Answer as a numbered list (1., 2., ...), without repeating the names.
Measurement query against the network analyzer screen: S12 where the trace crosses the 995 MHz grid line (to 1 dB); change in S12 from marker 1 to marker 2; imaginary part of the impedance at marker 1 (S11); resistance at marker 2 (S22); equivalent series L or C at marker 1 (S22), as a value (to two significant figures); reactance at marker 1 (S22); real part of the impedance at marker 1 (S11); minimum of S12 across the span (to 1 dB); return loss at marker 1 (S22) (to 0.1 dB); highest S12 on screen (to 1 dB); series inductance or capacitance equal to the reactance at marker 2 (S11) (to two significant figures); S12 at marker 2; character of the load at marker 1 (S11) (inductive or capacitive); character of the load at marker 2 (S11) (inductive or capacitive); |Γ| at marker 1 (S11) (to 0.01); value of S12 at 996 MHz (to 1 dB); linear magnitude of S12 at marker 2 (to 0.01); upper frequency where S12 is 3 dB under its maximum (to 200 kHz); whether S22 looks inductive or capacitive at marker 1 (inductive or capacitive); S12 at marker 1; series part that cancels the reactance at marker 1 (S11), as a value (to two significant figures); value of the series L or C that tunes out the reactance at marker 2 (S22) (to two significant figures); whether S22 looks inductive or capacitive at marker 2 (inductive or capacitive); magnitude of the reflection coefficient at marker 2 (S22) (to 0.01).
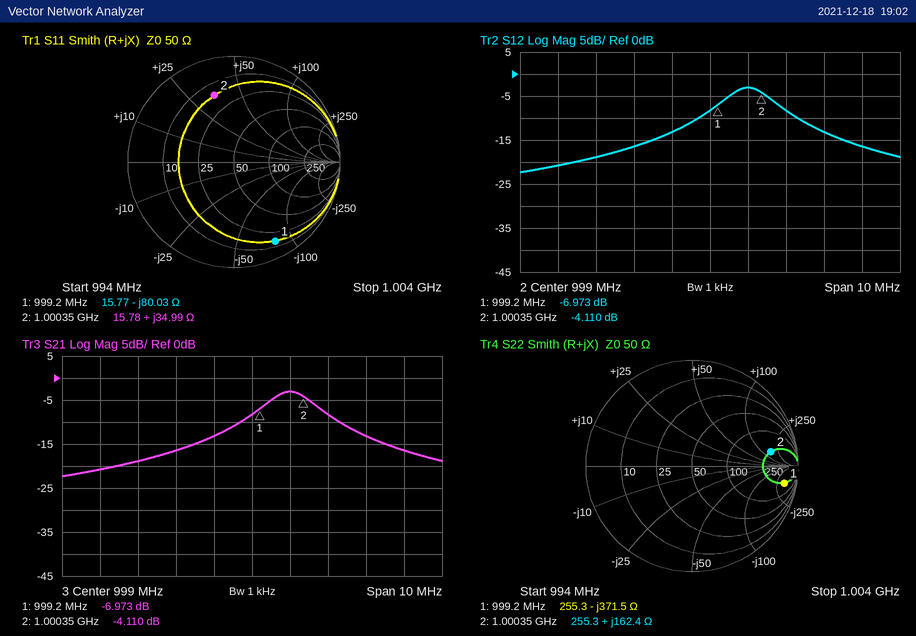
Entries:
1. -21 dB
2. 2.863 dB
3. -80.03 Ω
4. 255.3 Ω
5. 430 fF
6. -371.5 Ω
7. 15.77 Ω
8. -22 dB
9. 1.1 dB
10. -3 dB
11. 5.6 nH
12. -4.110 dB
13. capacitive
14. inductive
15. 0.84
16. -19 dB
17. 0.62
18. 1.0006 GHz
19. capacitive
20. -6.973 dB
21. 13 nH
22. 980 fF
23. inductive
24. 0.76
